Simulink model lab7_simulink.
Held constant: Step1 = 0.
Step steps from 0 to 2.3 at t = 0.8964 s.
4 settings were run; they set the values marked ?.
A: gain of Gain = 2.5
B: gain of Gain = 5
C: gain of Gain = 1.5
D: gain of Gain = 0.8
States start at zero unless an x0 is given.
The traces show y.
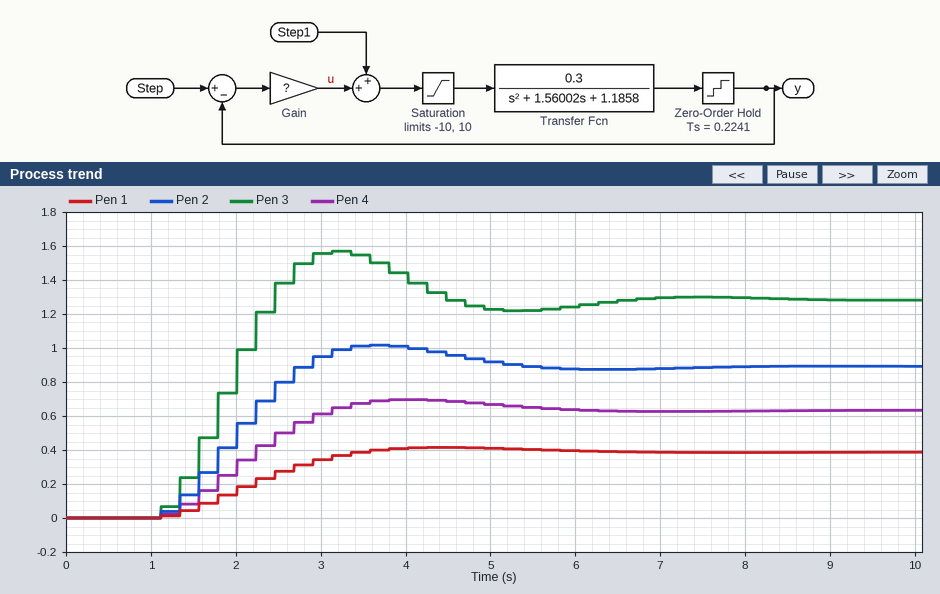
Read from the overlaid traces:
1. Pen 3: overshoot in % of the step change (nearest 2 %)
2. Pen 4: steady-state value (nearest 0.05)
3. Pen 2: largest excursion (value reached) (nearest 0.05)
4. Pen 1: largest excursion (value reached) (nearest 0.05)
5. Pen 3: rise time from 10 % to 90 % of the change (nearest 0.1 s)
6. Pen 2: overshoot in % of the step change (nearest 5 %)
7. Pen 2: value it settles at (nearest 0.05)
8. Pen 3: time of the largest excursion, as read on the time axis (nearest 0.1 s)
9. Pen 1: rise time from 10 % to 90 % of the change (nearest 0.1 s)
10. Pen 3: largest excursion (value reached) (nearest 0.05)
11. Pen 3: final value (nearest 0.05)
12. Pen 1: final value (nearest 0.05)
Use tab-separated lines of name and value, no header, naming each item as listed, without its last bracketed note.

Pen 3: overshoot in % of the step change	22 %
Pen 4: steady-state value	0.65
Pen 2: largest excursion (value reached)	1.00
Pen 1: largest excursion (value reached)	0.40
Pen 3: rise time from 10 % to 90 % of the change	0.9 s
Pen 2: overshoot in % of the step change	15 %
Pen 2: value it settles at	0.90
Pen 3: time of the largest excursion, as read on the time axis	3.1 s
Pen 1: rise time from 10 % to 90 % of the change	1.8 s
Pen 3: largest excursion (value reached)	1.55
Pen 3: final value	1.30
Pen 1: final value	0.40
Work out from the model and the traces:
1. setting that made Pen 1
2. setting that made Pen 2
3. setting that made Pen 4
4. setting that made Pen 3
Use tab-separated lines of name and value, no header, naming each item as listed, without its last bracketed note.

setting that made Pen 1	D
setting that made Pen 2	A
setting that made Pen 4	C
setting that made Pen 3	B
